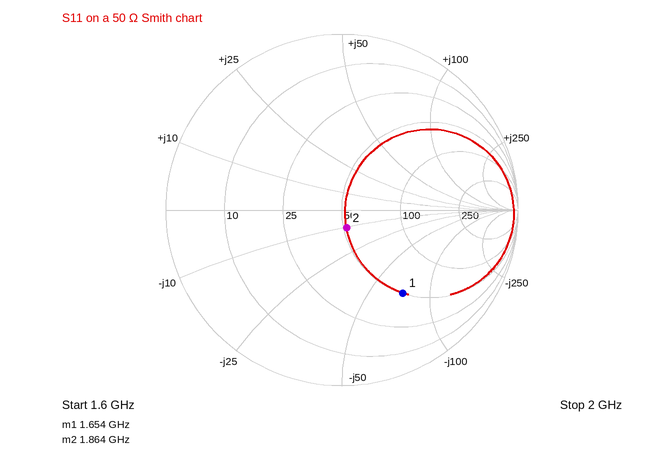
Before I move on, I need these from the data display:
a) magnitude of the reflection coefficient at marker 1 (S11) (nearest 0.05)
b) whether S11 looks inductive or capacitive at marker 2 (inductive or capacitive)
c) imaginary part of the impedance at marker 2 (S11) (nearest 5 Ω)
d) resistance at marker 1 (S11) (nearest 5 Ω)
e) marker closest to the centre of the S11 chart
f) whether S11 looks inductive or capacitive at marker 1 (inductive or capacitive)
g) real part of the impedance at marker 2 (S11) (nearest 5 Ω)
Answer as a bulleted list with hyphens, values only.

- 0.60
- capacitive
- -10 Ω
- 50 Ω
- marker 2
- capacitive
- 50 Ω
